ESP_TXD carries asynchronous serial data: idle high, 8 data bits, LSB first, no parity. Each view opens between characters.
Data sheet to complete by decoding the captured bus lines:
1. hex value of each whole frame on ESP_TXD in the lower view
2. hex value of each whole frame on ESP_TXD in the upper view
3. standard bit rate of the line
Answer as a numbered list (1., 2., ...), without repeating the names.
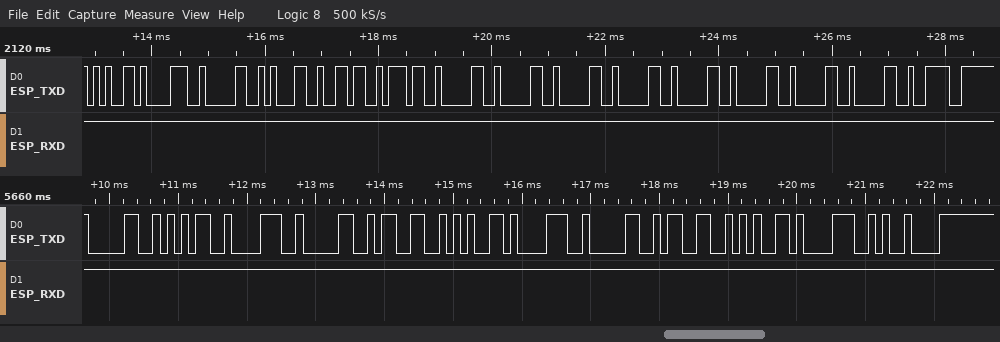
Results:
1. 30, 35, 38, 30, 33, 65, 38, 30, 33, 65, 38, 09
2. 65, 38, 30, 31, 36, 37, 30, 30, 30, 30, 30, 30, 30, 30, 9E
3. 9600 baud
